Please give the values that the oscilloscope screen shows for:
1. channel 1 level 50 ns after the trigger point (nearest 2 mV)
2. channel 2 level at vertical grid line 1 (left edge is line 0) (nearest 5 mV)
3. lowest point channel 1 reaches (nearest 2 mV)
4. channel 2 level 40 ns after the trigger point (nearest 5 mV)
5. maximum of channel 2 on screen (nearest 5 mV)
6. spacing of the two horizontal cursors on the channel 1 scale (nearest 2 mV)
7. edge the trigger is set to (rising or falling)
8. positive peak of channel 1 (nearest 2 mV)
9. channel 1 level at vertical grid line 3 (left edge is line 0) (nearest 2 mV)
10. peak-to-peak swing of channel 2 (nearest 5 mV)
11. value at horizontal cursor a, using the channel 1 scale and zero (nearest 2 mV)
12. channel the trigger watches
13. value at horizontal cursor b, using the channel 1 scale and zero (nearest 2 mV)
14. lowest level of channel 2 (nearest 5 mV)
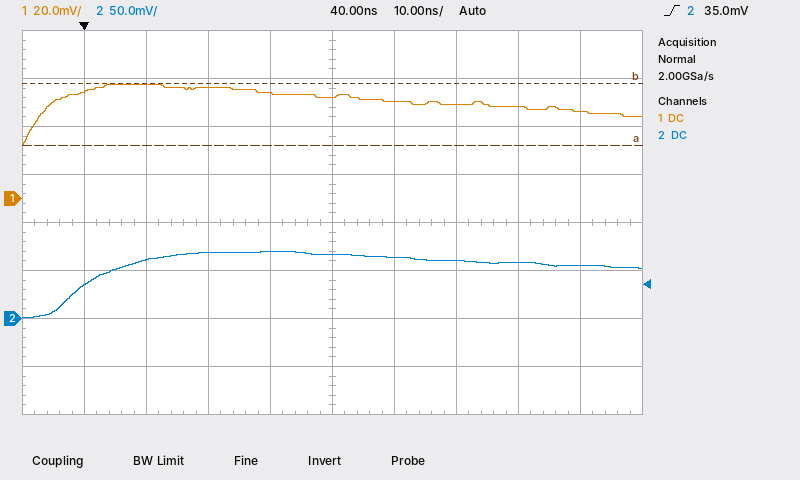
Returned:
40 mV
35 mV
22 mV
65 mV
70 mV
26 mV
rising
48 mV
46 mV
70 mV
22 mV
channel 2
48 mV
0 mV
